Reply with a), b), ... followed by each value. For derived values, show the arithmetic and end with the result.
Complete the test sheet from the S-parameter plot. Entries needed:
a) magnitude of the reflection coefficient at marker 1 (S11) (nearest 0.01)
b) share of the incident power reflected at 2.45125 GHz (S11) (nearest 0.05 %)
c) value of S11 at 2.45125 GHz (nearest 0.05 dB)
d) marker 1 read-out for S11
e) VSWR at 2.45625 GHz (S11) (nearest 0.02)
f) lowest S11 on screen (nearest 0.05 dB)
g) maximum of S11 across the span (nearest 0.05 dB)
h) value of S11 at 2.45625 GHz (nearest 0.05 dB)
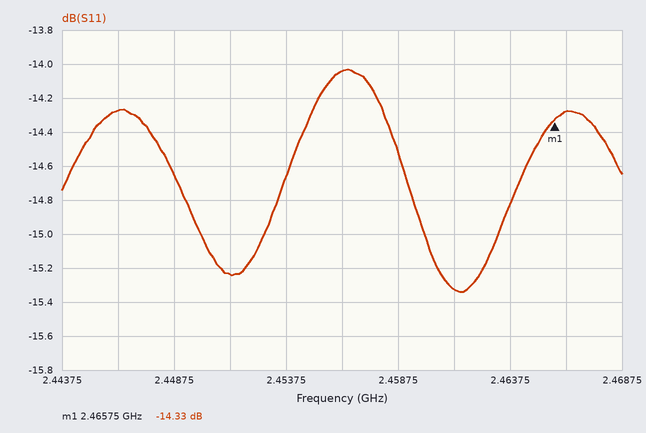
a) 10^(-14.33/20) ≈ 0.19
b) 10^(-15.25/10) ≈ 2.99 %, so 3.00 % to the nearest 0.05 %
c) -15.25 dB
d) -14.33 dB
e) |Γ| = 10^(-14.05/20) = 0.1984; VSWR = (1 + 0.1984)/(1 − 0.1984) ≈ 1.49, so 1.50 to the nearest 0.02
f) -15.35 dB
g) -14.05 dB
h) -14.05 dB
